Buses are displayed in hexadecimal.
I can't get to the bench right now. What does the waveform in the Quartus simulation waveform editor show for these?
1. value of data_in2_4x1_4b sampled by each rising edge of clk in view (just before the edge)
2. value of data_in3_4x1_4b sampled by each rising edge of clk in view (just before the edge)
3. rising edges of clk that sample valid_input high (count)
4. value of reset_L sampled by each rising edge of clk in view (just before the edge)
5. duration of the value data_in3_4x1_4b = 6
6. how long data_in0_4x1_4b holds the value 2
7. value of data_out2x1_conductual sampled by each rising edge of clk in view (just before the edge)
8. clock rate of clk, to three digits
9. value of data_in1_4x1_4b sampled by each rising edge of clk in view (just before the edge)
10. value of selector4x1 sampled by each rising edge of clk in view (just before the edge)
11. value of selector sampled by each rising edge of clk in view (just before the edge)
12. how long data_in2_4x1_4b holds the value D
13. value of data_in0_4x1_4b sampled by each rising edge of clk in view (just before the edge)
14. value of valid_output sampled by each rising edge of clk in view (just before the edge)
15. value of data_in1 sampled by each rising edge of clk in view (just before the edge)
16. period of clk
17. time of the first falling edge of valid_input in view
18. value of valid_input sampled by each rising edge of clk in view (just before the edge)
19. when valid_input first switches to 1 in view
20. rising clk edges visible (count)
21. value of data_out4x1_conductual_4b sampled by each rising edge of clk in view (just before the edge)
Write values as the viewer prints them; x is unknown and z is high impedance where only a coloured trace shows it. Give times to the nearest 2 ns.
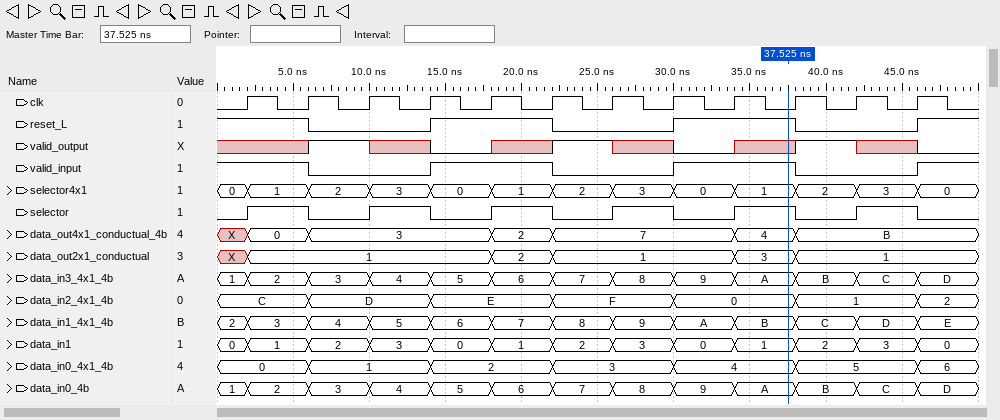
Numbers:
C, C, D, D, E, E, F, F, 0, 0, 1, 1
1, 2, 3, 4, 5, 6, 7, 8, 9, A, B, C
6
1 1 0 0 1 1 0 0 1 1 0 0
4 ns
8 ns
X, 1, 1, 1, 1, 2, 1, 1, 1, 3, 1, 1
250 MHz
2, 3, 4, 5, 6, 7, 8, 9, A, B, C, D
0, 1, 2, 3, 0, 1, 2, 3, 0, 1, 2, 3
0 1 0 1 0 1 0 1 0 1 0 1
8 ns
0, 0, 1, 1, 2, 2, 3, 3, 4, 4, 5, 5
x x 1 x 0 x 1 x 0 x 1 x
0, 1, 2, 3, 0, 1, 2, 3, 0, 1, 2, 3
4 ns
6 ns
1 1 0 0 1 1 0 0 1 1 0 0
14 ns
12
X, 0, 3, 3, 3, 2, 7, 7, 7, 4, B, B
